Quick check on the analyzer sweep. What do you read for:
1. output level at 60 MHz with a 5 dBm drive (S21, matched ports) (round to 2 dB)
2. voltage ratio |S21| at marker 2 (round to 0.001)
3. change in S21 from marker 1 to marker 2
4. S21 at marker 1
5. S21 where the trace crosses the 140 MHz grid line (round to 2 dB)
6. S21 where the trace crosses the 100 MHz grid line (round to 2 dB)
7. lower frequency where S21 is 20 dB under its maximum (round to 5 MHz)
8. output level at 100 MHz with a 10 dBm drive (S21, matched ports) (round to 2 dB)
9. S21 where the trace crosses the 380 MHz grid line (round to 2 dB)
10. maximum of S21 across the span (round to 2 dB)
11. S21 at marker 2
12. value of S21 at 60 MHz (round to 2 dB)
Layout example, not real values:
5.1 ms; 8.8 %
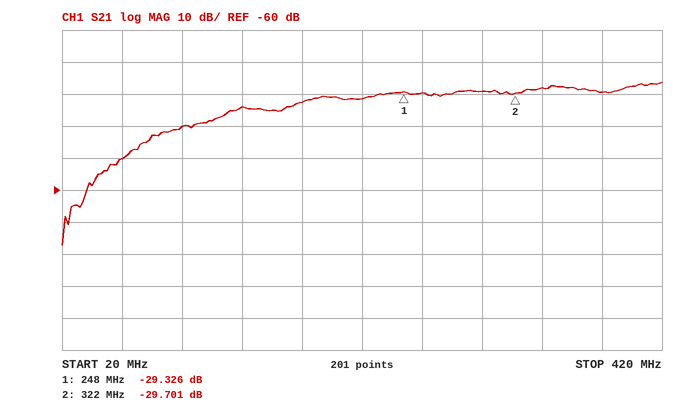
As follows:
-46 dBm; 0.033; -0.375 dB; -29.326 dB; -34 dB; -40 dB; 70 MHz; -30 dBm; -30 dB; -26 dB; -29.701 dB; -50 dB
